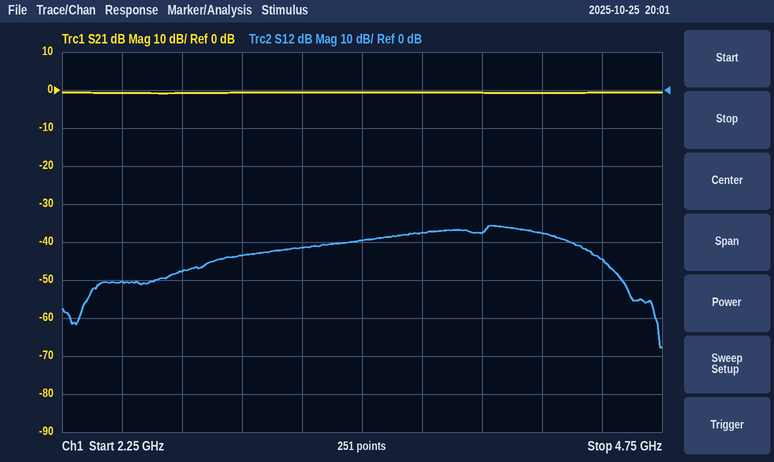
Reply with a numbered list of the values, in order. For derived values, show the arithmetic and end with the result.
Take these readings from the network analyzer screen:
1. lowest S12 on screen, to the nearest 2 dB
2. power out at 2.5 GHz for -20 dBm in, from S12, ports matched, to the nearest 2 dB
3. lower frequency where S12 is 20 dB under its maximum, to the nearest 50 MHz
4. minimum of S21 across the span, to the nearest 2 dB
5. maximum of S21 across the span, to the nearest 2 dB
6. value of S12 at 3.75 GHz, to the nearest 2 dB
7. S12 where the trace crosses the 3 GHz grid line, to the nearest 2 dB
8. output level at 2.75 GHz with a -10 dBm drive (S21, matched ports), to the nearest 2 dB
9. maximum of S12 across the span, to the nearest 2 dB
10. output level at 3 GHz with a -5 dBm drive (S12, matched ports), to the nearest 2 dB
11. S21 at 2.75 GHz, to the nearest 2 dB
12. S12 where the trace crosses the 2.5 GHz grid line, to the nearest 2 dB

1. -68 dB
2. -20 dBm + (-50 dB) = -70 dBm
3. 2.35 GHz
4. 0 dB
5. 0 dB
6. -38 dB
7. -44 dB
8. -10 dBm + (0 dB) = -10 dBm
9. -36 dB
10. -5 dBm + (-44 dB) = -48 dBm
11. 0 dB
12. -50 dB
